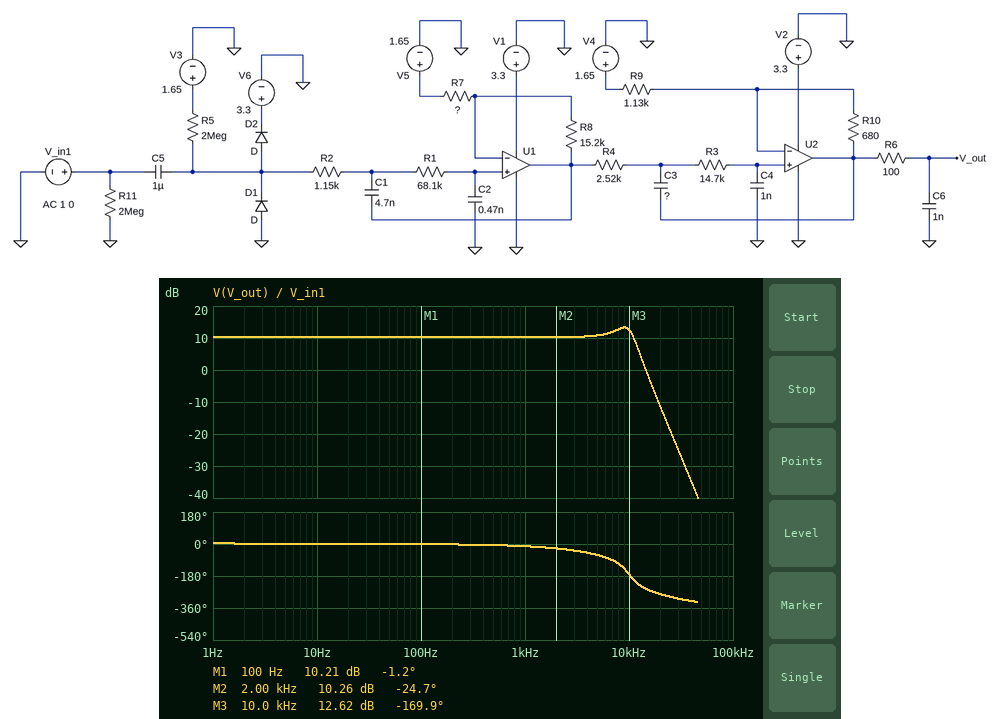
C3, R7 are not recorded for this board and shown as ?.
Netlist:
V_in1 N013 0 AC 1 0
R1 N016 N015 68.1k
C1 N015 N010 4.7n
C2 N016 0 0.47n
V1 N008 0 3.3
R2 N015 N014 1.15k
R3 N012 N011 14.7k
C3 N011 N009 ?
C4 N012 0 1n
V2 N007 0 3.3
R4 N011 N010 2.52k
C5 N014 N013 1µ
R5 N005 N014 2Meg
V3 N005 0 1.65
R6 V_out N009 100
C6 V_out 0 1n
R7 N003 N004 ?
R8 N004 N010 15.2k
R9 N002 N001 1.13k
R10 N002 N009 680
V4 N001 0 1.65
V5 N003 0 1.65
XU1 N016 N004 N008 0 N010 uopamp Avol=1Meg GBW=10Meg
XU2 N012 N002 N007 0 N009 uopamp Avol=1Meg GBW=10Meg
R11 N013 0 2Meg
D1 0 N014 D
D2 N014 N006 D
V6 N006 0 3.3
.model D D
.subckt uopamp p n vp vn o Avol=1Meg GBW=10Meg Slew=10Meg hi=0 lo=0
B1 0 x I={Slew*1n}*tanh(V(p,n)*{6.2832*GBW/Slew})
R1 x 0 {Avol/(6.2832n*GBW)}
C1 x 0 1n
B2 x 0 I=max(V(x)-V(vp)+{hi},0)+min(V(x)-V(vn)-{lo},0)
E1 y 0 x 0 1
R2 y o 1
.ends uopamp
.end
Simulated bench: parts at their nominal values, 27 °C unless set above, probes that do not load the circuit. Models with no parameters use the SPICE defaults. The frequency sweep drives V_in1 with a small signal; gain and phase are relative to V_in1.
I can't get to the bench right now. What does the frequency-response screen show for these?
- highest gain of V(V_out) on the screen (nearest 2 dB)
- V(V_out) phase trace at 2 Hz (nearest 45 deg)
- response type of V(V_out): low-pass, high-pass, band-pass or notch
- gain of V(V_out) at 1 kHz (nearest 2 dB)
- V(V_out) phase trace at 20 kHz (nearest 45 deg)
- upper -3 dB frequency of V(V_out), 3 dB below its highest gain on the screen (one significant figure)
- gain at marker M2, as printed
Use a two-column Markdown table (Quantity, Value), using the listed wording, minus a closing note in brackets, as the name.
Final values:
| Quantity | Value |
|---|---|
| highest gain of V(V_out) on the screen | 14 dB |
| V(V_out) phase trace at 2 Hz | 0 deg |
| response type of V(V_out): low-pass, high-pass, band-pass or notch | low-pass |
| gain of V(V_out) at 1 kHz | 10 dB |
| V(V_out) phase trace at 20 kHz | -270 deg |
| upper -3 dB frequency of V(V_out), 3 dB below its highest gain on the screen | 10 kHz |
| gain at marker M2, as printed | 10.26 dB |
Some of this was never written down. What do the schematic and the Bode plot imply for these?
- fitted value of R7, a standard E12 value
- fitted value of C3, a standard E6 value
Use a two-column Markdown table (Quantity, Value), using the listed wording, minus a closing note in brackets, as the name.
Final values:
| Quantity | Value |
|---|---|
| fitted value of R7, a standard E12 value | 15 kΩ |
| fitted value of C3, a standard E6 value | 6.8 nF |
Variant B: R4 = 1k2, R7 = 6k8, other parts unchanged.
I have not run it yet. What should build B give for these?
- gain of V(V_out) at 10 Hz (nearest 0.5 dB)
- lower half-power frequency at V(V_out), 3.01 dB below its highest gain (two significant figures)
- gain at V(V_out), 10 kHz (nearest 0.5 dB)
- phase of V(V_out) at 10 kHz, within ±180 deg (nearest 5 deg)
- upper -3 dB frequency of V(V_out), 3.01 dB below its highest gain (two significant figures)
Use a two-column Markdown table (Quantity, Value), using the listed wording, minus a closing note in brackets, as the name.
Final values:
| Quantity | Value |
|---|---|
| gain of V(V_out) at 10 Hz | 14.5 dB |
| lower half-power frequency at V(V_out), 3.01 dB below its highest gain | 81 mHz |
| gain at V(V_out), 10 kHz | 13.0 dB |
| phase of V(V_out) at 10 kHz, within ±180 deg | -130 deg |
| upper -3 dB frequency of V(V_out), 3.01 dB below its highest gain | 12 kHz |
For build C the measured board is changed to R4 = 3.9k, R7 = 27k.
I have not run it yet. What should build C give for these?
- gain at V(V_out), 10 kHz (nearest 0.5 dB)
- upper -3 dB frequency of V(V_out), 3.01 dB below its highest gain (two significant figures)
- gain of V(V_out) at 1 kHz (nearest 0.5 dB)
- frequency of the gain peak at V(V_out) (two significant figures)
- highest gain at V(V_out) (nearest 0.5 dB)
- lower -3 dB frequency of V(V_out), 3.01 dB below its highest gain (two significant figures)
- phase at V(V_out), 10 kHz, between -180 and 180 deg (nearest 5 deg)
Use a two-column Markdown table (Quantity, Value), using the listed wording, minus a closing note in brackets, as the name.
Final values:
| Quantity | Value |
|---|---|
| gain at V(V_out), 10 kHz | 7.5 dB |
| upper -3 dB frequency of V(V_out), 3.01 dB below its highest gain | 8.5 kHz |
| gain of V(V_out) at 1 kHz | 8.0 dB |
| frequency of the gain peak at V(V_out) | 8.0 kHz |
| highest gain at V(V_out) | 21.5 dB |
| lower -3 dB frequency of V(V_out), 3.01 dB below its highest gain | 7.4 kHz |
| phase at V(V_out), 10 kHz, between -180 and 180 deg | 115 deg |
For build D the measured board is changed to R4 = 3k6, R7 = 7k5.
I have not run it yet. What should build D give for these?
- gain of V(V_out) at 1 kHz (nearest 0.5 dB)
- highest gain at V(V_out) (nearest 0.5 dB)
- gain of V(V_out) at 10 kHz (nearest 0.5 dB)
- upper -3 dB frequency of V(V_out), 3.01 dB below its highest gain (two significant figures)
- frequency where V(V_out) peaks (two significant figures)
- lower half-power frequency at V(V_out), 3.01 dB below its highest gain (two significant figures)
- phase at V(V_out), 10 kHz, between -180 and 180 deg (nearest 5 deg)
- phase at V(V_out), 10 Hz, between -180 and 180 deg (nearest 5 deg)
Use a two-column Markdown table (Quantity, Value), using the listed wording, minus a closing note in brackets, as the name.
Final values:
| Quantity | Value |
|---|---|
| gain of V(V_out) at 1 kHz | 14.0 dB |
| highest gain at V(V_out) | 26.5 dB |
| gain of V(V_out) at 10 kHz | 17.0 dB |
| upper -3 dB frequency of V(V_out), 3.01 dB below its highest gain | 9.0 kHz |
| frequency where V(V_out) peaks | 8.3 kHz |
| lower half-power frequency at V(V_out), 3.01 dB below its highest gain | 7.4 kHz |
| phase at V(V_out), 10 kHz, between -180 and 180 deg | 130 deg |
| phase at V(V_out), 10 Hz, between -180 and 180 deg | 0 deg |
